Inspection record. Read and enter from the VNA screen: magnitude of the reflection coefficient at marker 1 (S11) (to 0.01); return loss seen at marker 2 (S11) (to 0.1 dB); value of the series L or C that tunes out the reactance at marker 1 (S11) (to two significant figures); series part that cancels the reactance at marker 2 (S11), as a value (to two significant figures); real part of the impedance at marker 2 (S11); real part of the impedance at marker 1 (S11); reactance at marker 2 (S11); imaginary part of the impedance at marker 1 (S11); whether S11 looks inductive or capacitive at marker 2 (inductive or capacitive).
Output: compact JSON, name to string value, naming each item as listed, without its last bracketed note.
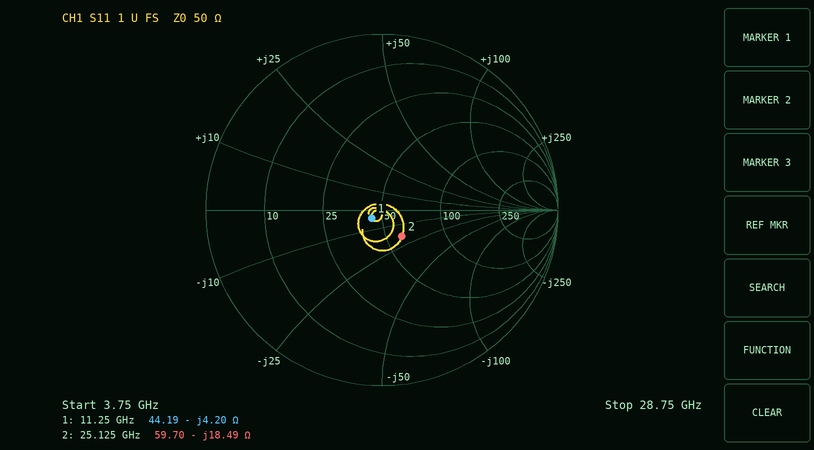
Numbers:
{"magnitude of the reflection coefficient at marker 1 (S11)": "0.08", "return loss seen at marker 2 (S11)": "14.5 dB", "value of the series L or C that tunes out the reactance at marker 1 (S11)": "59 pH", "series part that cancels the reactance at marker 2 (S11), as a value": "120 pH", "real part of the impedance at marker 2": "59.70 Ω", "real part of the impedance at marker 1": "44.19 Ω", "reactance at marker 2": "-18.49 Ω", "imaginary part of the impedance at marker 1": "-4.20 Ω", "whether S11 looks inductive or capacitive at marker 2": "capacitive"}
